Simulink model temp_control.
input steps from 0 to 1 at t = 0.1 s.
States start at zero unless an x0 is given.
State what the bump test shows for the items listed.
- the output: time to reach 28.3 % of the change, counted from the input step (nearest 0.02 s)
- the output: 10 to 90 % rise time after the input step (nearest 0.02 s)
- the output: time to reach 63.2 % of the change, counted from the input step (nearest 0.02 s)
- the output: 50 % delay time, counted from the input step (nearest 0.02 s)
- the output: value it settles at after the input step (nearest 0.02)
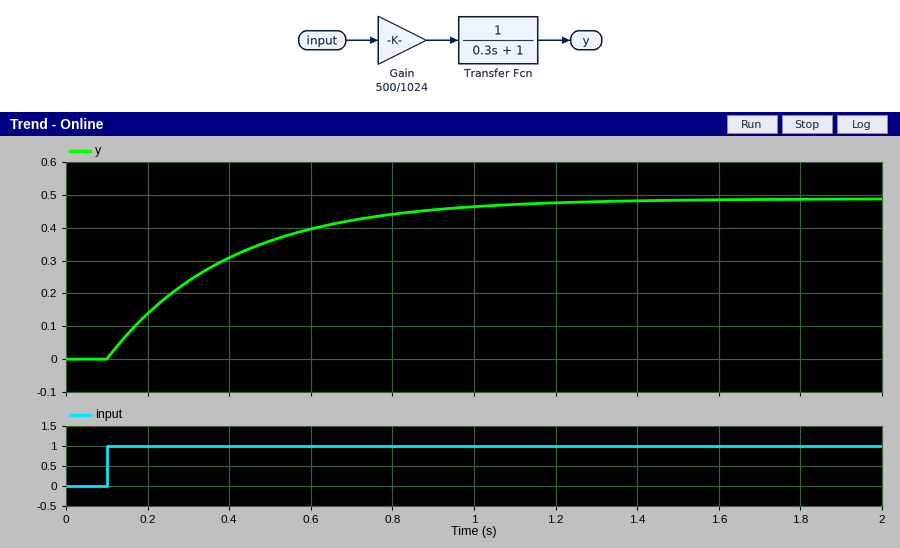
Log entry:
0.10 s
0.66 s
0.30 s
0.20 s
0.48
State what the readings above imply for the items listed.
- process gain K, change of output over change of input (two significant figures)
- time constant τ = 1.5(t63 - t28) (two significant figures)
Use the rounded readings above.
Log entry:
0.48
0.30 s
